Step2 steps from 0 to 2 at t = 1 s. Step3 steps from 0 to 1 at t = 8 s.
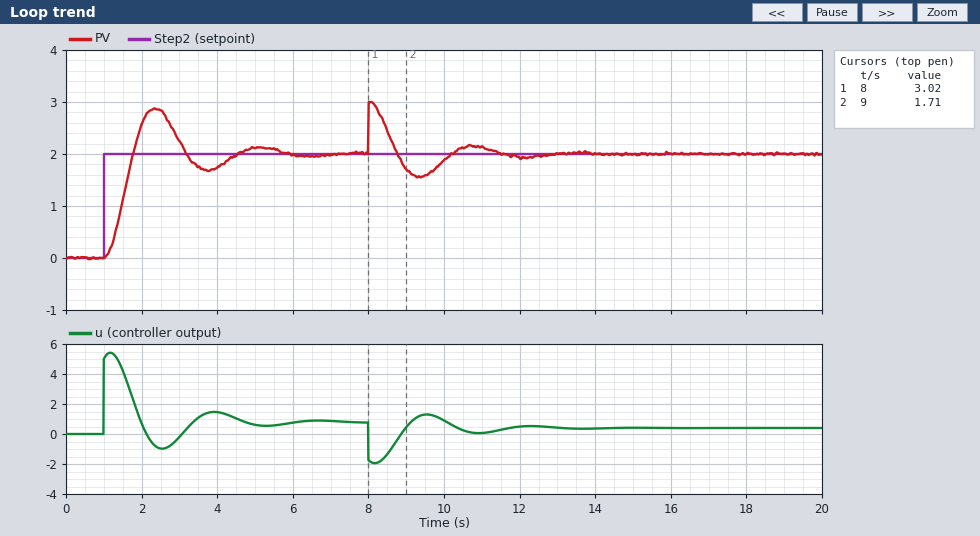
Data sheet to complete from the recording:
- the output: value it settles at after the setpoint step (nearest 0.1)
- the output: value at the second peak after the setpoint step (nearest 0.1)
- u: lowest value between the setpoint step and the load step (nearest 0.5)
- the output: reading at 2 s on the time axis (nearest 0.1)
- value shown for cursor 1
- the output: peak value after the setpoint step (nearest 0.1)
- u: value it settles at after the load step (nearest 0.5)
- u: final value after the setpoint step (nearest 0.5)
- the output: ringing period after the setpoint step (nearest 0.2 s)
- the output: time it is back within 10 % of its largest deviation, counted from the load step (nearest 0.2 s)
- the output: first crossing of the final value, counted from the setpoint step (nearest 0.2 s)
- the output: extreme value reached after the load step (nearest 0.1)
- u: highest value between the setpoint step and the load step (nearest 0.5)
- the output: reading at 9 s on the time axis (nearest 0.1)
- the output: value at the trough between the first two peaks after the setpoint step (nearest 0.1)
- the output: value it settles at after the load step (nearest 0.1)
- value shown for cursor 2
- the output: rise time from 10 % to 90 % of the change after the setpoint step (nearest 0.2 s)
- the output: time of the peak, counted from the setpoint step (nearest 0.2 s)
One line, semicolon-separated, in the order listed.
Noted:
2.0; 2.1; -1.0; 2.6; 3.02; 2.9; 0.5; 1.0; 2.8 s; 3.2 s; 0.8 s; 3.0; 5.5; 1.7; 1.7; 2.0; 1.71; 0.6 s; 1.4 s
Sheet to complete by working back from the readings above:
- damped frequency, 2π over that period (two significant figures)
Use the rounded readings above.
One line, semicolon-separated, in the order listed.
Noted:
2.2 rad/s
